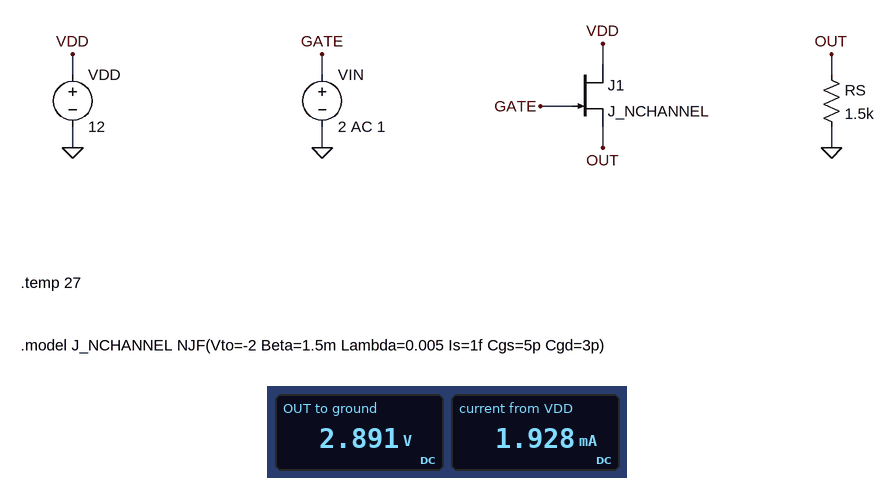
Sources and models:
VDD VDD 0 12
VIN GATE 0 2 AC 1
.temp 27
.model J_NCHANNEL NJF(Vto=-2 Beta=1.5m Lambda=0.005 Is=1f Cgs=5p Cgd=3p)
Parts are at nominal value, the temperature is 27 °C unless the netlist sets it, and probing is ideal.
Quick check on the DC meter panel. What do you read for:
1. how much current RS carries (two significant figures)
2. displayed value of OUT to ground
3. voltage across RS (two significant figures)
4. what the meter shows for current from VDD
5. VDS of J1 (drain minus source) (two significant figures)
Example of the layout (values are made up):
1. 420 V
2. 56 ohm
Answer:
1. 1.9 mA
2. 2.891 V
3. 2.9 V
4. 1.928 mA
5. 9.1 V
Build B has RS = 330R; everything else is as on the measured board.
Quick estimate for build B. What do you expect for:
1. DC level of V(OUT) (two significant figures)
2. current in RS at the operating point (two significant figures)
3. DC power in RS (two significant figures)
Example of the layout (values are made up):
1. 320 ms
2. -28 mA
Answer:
1. 2.0 V
2. 6.1 mA
3. 12 mW
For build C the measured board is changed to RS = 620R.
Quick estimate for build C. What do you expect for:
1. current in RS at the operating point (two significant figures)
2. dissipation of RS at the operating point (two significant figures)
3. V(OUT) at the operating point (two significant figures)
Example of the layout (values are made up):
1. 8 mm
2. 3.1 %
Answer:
1. 3.9 mA
2. 9.5 mW
3. 2.4 V
